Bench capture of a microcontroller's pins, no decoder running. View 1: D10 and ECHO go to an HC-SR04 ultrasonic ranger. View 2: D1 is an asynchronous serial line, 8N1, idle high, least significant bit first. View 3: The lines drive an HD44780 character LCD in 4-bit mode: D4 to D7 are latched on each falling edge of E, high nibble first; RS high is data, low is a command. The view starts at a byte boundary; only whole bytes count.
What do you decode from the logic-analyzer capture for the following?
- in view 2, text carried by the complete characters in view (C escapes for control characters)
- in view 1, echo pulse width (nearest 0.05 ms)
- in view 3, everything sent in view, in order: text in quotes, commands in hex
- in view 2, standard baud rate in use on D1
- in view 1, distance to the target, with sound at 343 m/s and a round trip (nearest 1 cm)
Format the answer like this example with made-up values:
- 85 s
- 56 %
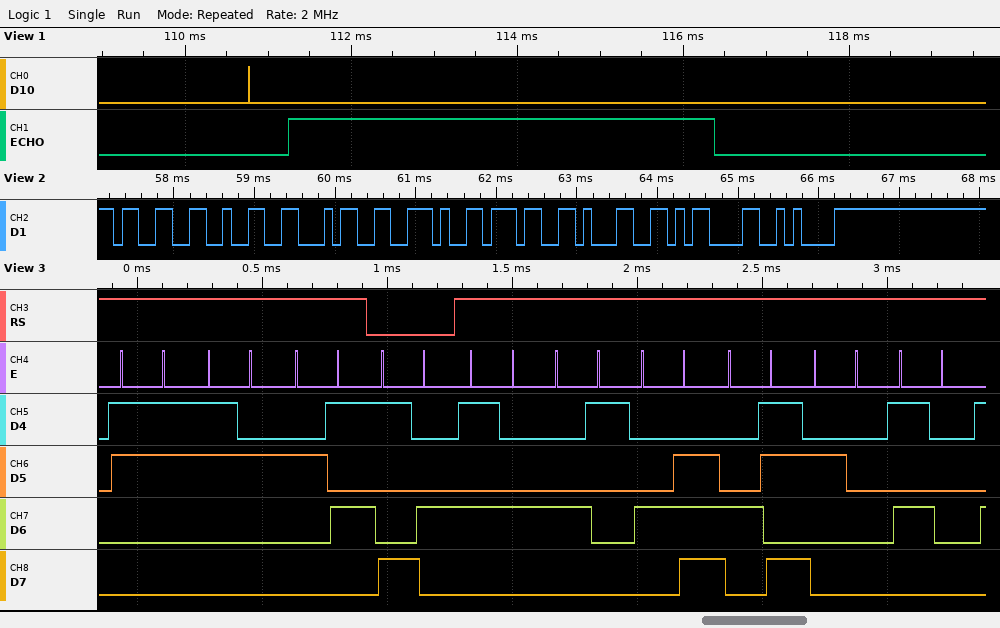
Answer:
- "324.71\r\n"
- 5.15 ms
- "32%" 0x94 "TANK P"
- 9600 baud
- 88 cm
